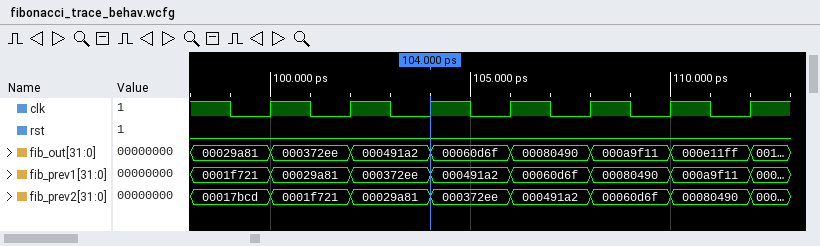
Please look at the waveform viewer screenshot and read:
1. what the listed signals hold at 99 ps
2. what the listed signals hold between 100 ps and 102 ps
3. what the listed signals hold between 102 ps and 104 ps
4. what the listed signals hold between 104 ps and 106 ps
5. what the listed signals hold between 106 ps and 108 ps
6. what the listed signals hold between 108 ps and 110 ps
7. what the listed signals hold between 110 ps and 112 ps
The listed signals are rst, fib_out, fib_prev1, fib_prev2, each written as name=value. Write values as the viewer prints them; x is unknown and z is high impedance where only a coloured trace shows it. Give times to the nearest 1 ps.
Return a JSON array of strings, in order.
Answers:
["rst=0, fib_out=00029a81, fib_prev1=0001f721, fib_prev2=00017bcd", "rst=0, fib_out=000372ee, fib_prev1=00029a81, fib_prev2=0001f721", "rst=0, fib_out=000491a2, fib_prev1=000372ee, fib_prev2=00029a81", "rst=0, fib_out=00060d6f, fib_prev1=000491a2, fib_prev2=000372ee", "rst=0, fib_out=00080490, fib_prev1=00060d6f, fib_prev2=000491a2", "rst=0, fib_out=000a9f11, fib_prev1=00080490, fib_prev2=00060d6f", "rst=0, fib_out=000e11ff, fib_prev1=000a9f11, fib_prev2=00080490"]
